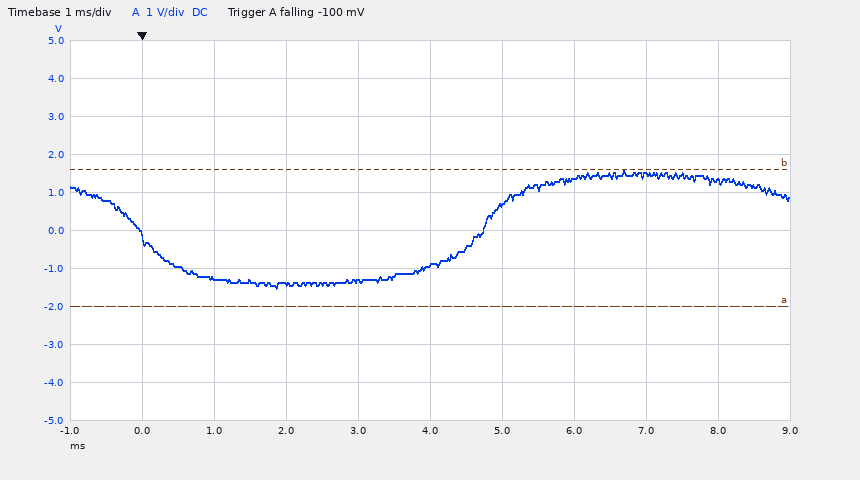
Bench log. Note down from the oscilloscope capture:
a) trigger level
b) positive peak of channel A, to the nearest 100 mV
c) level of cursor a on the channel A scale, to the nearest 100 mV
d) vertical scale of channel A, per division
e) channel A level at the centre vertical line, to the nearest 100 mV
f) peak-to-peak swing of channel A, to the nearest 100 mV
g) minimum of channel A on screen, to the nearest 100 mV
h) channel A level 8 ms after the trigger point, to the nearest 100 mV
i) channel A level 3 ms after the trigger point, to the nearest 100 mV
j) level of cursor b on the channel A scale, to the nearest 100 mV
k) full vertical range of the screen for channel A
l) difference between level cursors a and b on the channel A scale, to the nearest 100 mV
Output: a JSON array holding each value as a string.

["-100 mV", "1.6 V", "-2.0 V", "1 V", "-900 mV", "3.1 V", "-1.5 V", "1.3 V", "-1.3 V", "1.6 V", "10 V", "3.6 V"]
